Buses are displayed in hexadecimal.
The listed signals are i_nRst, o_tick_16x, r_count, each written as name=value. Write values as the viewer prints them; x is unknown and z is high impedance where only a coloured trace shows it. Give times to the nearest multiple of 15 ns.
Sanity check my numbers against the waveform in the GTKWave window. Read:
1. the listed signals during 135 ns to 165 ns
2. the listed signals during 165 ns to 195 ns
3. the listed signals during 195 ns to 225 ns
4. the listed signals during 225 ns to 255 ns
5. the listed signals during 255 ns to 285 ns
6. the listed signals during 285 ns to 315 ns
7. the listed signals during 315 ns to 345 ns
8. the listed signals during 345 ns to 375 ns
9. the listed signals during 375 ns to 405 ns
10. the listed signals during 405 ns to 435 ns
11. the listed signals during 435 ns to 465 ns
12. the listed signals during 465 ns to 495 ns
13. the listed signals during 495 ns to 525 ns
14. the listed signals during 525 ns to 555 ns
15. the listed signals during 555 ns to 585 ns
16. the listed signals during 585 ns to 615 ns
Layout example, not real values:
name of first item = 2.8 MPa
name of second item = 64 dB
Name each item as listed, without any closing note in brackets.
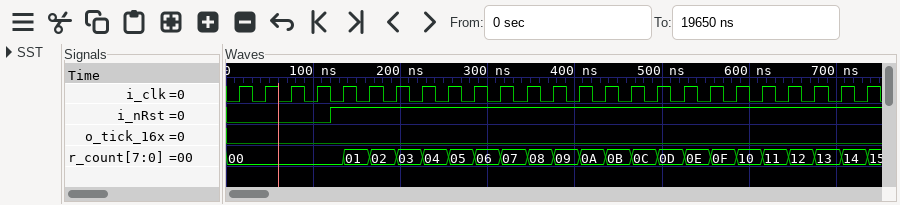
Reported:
the listed signals during 135 ns to 165 ns = i_nRst=1, o_tick_16x=0, r_count=01
the listed signals during 165 ns to 195 ns = i_nRst=1, o_tick_16x=0, r_count=02
the listed signals during 195 ns to 225 ns = i_nRst=1, o_tick_16x=0, r_count=03
the listed signals during 225 ns to 255 ns = i_nRst=1, o_tick_16x=0, r_count=04
the listed signals during 255 ns to 285 ns = i_nRst=1, o_tick_16x=0, r_count=05
the listed signals during 285 ns to 315 ns = i_nRst=1, o_tick_16x=0, r_count=06
the listed signals during 315 ns to 345 ns = i_nRst=1, o_tick_16x=0, r_count=07
the listed signals during 345 ns to 375 ns = i_nRst=1, o_tick_16x=0, r_count=08
the listed signals during 375 ns to 405 ns = i_nRst=1, o_tick_16x=0, r_count=09
the listed signals during 405 ns to 435 ns = i_nRst=1, o_tick_16x=0, r_count=0A
the listed signals during 435 ns to 465 ns = i_nRst=1, o_tick_16x=0, r_count=0B
the listed signals during 465 ns to 495 ns = i_nRst=1, o_tick_16x=0, r_count=0C
the listed signals during 495 ns to 525 ns = i_nRst=1, o_tick_16x=0, r_count=0D
the listed signals during 525 ns to 555 ns = i_nRst=1, o_tick_16x=0, r_count=0E
the listed signals during 555 ns to 585 ns = i_nRst=1, o_tick_16x=0, r_count=0F
the listed signals during 585 ns to 615 ns = i_nRst=1, o_tick_16x=0, r_count=10
